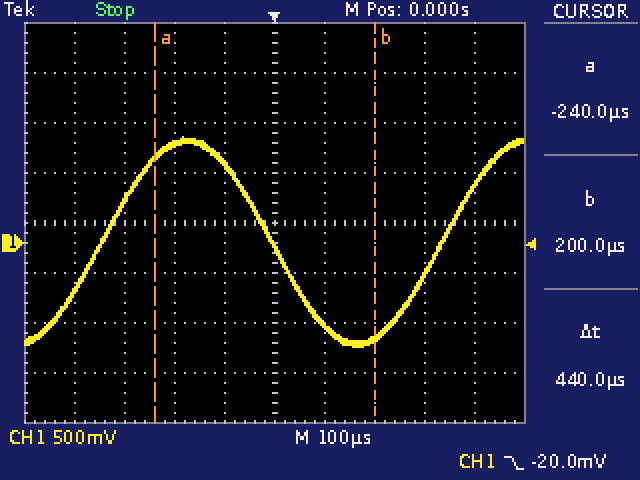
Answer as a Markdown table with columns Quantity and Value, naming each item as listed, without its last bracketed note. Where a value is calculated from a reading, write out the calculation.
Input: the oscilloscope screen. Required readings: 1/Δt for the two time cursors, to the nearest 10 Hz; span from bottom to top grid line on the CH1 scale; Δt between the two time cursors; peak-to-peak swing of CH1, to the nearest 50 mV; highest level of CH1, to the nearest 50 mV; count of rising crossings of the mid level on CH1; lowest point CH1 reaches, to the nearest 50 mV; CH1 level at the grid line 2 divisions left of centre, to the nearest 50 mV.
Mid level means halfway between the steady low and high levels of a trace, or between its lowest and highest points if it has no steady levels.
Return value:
| Quantity | Value |
|---|---|
| 1/Δt for the two time cursors, to the nearest 10 Hz | 1 / 440 µs ≈ 2.27 kHz |
| span from bottom to top grid line on the CH1 scale | 4 V |
| Δt between the two time cursors | 440 µs |
| peak-to-peak swing of CH1, to the nearest 50 mV | 1.05 V − (-1.05 V) = 2.10 V |
| highest level of CH1, to the nearest 50 mV | 1.05 V |
| count of rising crossings of the mid level on CH1 | 2 |
| lowest point CH1 reaches, to the nearest 50 mV | -1.05 V |
| CH1 level at the grid line 2 divisions left of centre, to the nearest 50 mV | 1.00 V |
